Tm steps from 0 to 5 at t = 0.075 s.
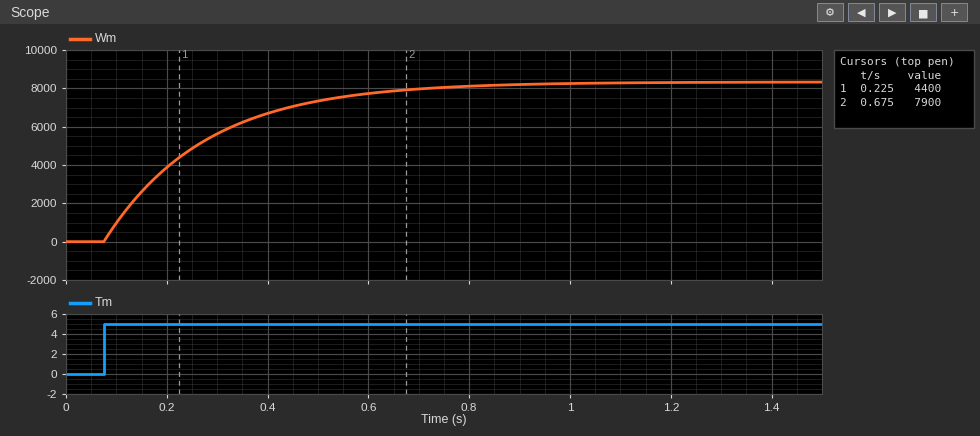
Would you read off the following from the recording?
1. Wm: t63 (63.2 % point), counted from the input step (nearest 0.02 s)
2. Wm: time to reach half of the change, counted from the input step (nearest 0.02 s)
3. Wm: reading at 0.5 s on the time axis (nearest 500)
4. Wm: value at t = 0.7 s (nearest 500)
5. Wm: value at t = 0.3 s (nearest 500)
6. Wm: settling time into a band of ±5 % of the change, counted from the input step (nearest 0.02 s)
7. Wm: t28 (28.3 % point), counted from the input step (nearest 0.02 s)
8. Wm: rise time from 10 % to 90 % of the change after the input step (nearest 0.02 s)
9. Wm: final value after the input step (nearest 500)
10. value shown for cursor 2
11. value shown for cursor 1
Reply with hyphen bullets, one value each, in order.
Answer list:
- 0.20 s
- 0.14 s
- 7500
- 8000
- 5500
- 0.60 s
- 0.06 s
- 0.44 s
- 8500
- 7900
- 4400
